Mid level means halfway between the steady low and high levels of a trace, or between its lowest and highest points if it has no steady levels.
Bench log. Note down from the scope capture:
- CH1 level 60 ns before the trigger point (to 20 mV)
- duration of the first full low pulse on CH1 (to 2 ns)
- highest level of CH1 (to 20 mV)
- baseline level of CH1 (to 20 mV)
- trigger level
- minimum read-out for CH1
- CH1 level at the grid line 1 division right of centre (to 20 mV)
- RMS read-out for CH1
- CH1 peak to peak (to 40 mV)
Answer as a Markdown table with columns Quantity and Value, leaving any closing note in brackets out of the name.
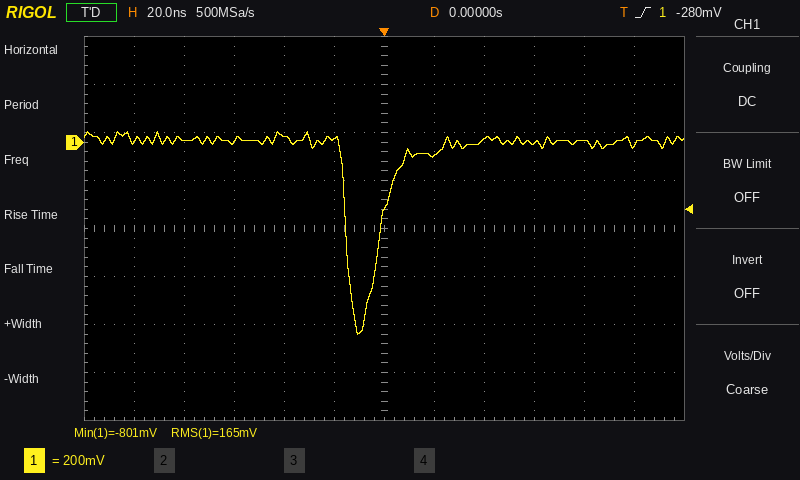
| Quantity | Value |
|---|---|
| CH1 level 60 ns before the trigger point | 0 mV |
| duration of the first full low pulse on CH1 | 14 ns |
| highest level of CH1 | 40 mV |
| baseline level of CH1 | 0 mV |
| trigger level | -280 mV |
| minimum read-out for CH1 | -801 mV |
| CH1 level at the grid line 1 division right of centre | -60 mV |
| RMS read-out for CH1 | 165 mV |
| CH1 peak to peak | 840 mV |
